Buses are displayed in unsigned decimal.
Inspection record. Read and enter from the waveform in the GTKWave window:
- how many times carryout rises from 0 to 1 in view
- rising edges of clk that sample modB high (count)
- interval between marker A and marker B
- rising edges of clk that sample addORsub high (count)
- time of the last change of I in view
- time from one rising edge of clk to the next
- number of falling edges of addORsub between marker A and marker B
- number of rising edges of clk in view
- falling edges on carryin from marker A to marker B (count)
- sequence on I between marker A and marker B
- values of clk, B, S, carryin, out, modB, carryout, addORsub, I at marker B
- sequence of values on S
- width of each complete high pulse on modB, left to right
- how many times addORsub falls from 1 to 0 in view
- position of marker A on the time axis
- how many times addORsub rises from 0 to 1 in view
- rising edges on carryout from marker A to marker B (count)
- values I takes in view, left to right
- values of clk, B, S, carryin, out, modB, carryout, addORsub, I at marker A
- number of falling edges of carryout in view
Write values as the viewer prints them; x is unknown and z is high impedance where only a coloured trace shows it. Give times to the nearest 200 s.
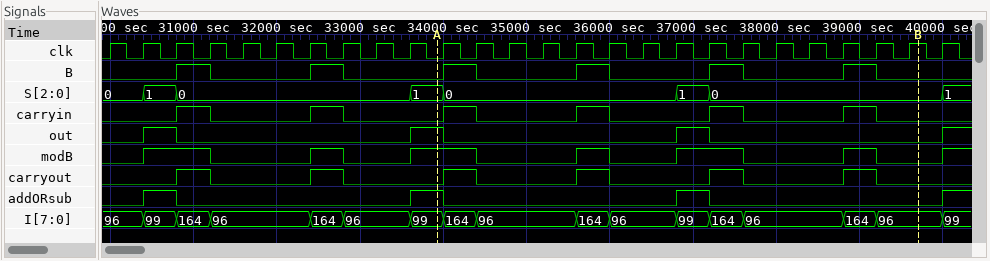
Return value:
6
9
5800 s
3
40000 s
400 s
2
26
4
99, 164, 96, 164, 96, 99, 164, 96, 164, 96
clk=1, B=0, S=0, carryin=0, out=0, modB=0, carryout=0, addORsub=0, I=96
0, 1, 0, 1, 0, 1, 0, 1
800 s, 400 s, 800 s, 400 s, 800 s, 400 s
3
34000 s
4
4
96, 99, 164, 96, 164, 96, 99, 164, 96, 164, 96, 99, 164, 96, 164, 96, 99
clk=0, B=0, S=1, carryin=0, out=1, modB=1, carryout=0, addORsub=1, I=99
6
